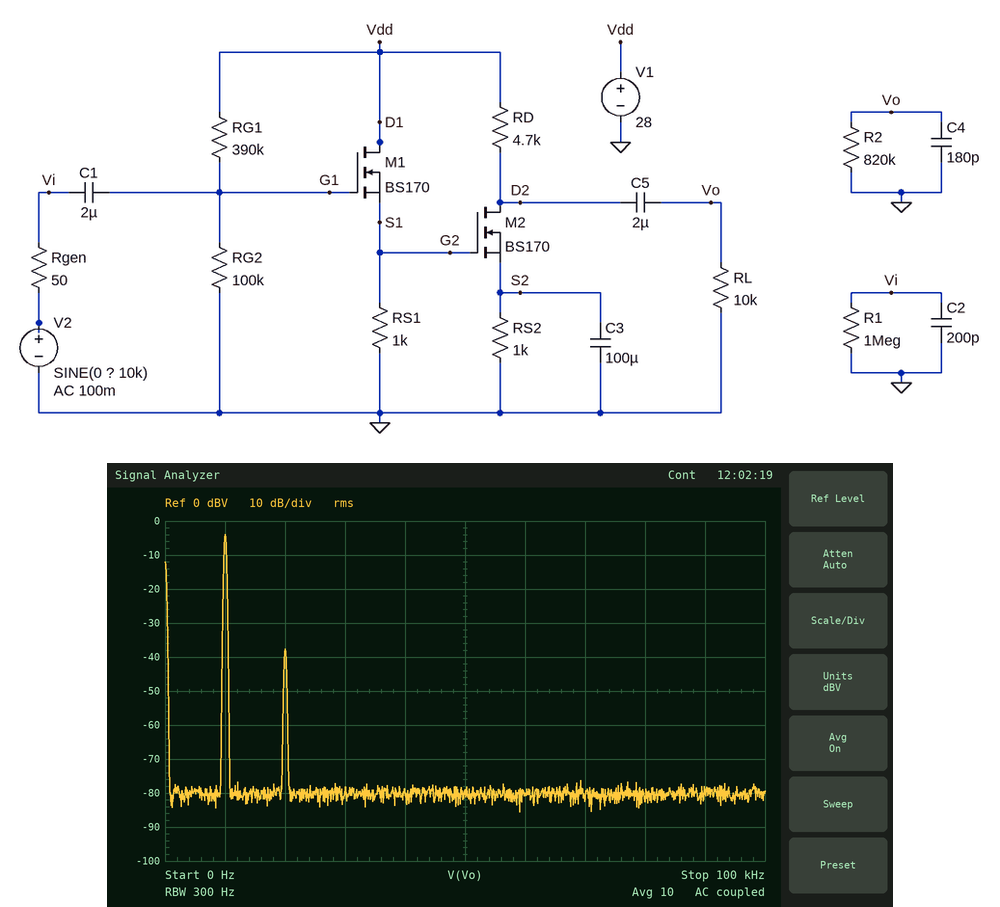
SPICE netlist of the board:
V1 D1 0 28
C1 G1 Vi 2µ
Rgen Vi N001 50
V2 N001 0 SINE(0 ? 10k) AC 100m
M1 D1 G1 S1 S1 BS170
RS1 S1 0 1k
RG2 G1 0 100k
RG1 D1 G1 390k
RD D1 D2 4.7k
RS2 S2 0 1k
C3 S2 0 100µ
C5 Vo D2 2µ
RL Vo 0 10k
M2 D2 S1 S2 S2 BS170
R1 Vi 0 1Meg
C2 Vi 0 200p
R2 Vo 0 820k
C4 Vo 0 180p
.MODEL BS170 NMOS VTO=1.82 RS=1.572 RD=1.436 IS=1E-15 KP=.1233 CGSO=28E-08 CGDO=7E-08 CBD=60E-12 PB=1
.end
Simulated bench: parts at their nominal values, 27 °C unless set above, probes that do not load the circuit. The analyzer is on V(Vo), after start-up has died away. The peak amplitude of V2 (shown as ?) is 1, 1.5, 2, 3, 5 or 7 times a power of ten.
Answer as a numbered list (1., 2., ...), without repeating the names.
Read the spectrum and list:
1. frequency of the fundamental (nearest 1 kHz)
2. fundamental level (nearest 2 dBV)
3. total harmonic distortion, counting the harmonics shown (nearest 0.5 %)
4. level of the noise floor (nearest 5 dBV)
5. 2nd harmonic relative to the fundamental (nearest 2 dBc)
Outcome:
1. 10 kHz
2. -4 dBV
3. 2.0 %
4. -80 dBV
5. -34 dBc
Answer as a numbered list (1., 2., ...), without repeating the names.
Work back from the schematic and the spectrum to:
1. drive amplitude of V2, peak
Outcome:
1. 15 mV
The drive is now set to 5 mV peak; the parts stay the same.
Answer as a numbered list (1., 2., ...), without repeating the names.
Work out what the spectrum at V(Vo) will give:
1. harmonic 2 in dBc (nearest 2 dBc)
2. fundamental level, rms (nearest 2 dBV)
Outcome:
1. -44 dBc
2. -14 dBV
